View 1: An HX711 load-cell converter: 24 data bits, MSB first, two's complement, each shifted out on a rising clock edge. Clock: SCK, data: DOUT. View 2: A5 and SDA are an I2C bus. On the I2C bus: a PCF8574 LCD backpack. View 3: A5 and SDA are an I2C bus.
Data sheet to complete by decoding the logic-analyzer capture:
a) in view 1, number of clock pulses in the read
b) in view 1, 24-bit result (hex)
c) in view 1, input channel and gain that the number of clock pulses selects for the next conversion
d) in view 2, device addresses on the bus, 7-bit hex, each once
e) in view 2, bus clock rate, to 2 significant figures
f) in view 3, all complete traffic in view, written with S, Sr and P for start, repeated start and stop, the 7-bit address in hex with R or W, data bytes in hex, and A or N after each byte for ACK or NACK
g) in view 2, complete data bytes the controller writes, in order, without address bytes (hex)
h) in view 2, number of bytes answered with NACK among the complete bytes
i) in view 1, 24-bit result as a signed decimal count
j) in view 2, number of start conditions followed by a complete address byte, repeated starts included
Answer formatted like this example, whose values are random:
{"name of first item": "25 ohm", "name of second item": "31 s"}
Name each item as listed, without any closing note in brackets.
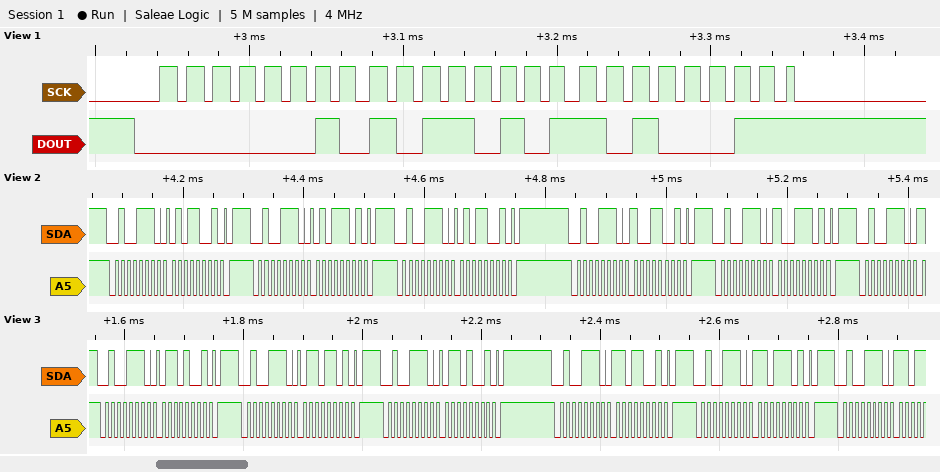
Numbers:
{"in view 1, number of clock pulses in the read": "25", "in view 1, 24-bit result": "0x02B5A3", "in view 1, input channel and gain that the number of clock pulses selects for the next conversion": "channel A, gain 128", "in view 2, device addresses on the bus, 7-bit hex, each once": "0x27", "in view 2, bus clock rate, to 2 significant figures": "100 kHz", "in view 3, all complete traffic in view, written with S, Sr and P for start, repeated start and stop, the 7-bit address in hex with R or W, data bytes in hex, and A or N after each byte for ACK or NACK": "S 27W A 69 A P S 27W A 6D A P S 27W A 69 A P S 27W A D9 A P S 27W A DD A P S 27W A", "in view 2, complete data bytes the controller writes, in order, without address bytes": "59 5D 59 99 9D", "in view 2, number of bytes answered with NACK among the complete bytes": "0", "in view 1, 24-bit result as a signed decimal count": "177571", "in view 2, number of start conditions followed by a complete address byte, repeated starts included": "6"}
